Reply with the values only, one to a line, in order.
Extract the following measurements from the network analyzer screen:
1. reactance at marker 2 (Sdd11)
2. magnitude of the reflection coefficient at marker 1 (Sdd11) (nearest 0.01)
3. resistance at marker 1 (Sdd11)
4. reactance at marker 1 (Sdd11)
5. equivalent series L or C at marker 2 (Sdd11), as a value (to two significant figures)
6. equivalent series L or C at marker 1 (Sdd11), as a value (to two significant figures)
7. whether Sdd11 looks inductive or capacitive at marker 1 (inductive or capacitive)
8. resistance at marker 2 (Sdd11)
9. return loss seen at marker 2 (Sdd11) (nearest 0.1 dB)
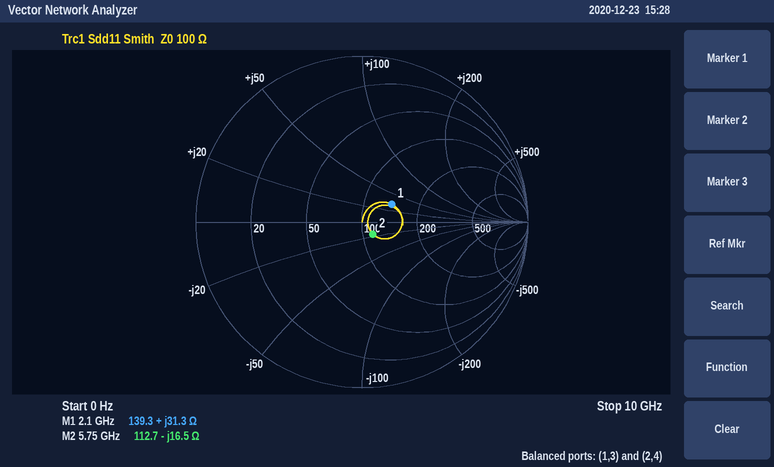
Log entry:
-16.5 Ω
0.21
139.3 Ω
+31.3 Ω
1.7 pF
2.4 nH
inductive
112.7 Ω
20.2 dB
